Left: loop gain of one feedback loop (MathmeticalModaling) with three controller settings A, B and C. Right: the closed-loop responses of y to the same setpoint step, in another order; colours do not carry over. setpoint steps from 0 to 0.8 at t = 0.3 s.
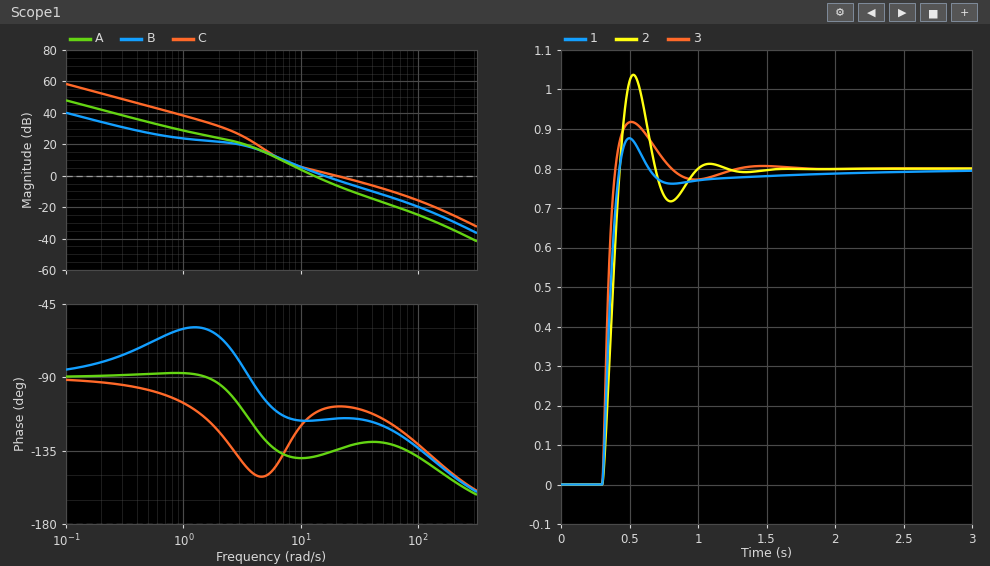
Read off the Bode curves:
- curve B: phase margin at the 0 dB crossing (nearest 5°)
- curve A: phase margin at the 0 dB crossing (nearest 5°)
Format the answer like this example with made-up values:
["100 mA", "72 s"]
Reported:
["65°", "40°"]
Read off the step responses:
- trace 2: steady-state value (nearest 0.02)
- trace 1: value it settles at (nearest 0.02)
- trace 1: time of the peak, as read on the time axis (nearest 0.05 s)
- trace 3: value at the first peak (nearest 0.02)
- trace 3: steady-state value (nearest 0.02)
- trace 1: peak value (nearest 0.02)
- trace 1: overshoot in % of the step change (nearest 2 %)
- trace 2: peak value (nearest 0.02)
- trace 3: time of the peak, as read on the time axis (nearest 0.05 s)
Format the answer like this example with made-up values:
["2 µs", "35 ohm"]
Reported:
["0.80", "0.80", "0.50 s", "0.92", "0.80", "0.88", "10 %", "1.04", "0.50 s"]
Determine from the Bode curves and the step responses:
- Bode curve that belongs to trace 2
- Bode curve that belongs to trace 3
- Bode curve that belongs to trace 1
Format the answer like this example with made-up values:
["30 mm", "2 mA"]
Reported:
["A", "C", "B"]
